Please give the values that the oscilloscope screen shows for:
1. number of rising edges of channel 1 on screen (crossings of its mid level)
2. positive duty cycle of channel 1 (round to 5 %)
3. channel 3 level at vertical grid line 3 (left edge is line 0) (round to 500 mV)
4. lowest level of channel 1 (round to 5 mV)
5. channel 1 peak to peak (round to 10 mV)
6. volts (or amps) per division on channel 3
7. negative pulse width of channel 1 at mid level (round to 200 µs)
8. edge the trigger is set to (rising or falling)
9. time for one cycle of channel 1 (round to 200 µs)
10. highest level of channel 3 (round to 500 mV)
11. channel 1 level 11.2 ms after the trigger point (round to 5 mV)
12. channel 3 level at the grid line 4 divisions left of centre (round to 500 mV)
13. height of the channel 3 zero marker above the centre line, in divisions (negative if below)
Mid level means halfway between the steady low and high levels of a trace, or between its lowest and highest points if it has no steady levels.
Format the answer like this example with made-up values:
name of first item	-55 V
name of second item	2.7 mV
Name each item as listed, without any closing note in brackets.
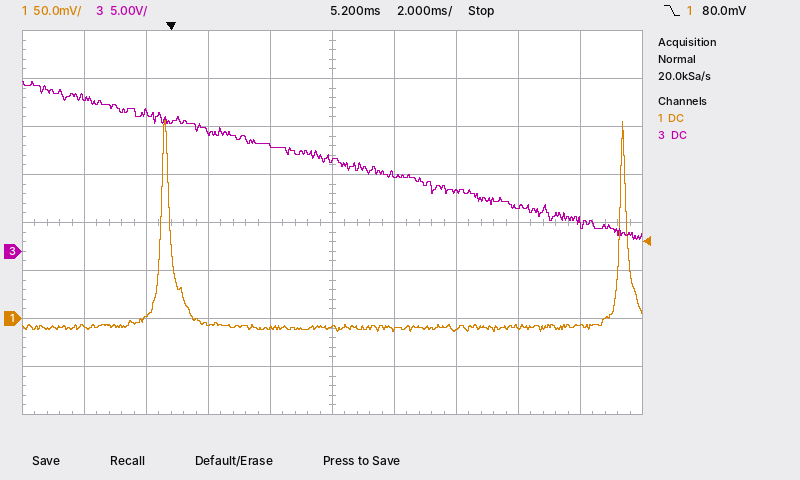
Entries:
number of rising edges of channel 1 on screen	2
positive duty cycle of channel 1	0 %
channel 3 level at vertical grid line 3 (left edge is line 0)	12.5 V
lowest level of channel 1	-15 mV
channel 1 peak to peak	220 mV
volts (or amps) per division on channel 3	5 V
negative pulse width of channel 1 at mid level	14.6 ms
edge the trigger is set to	falling
time for one cycle of channel 1	14.8 ms
highest level of channel 3	17.5 V
channel 1 level 11.2 ms after the trigger point	-10 mV
channel 3 level at the grid line 4 divisions left of centre	16.0 V
height of the channel 3 zero marker above the centre line, in divisions	-0.6 div
